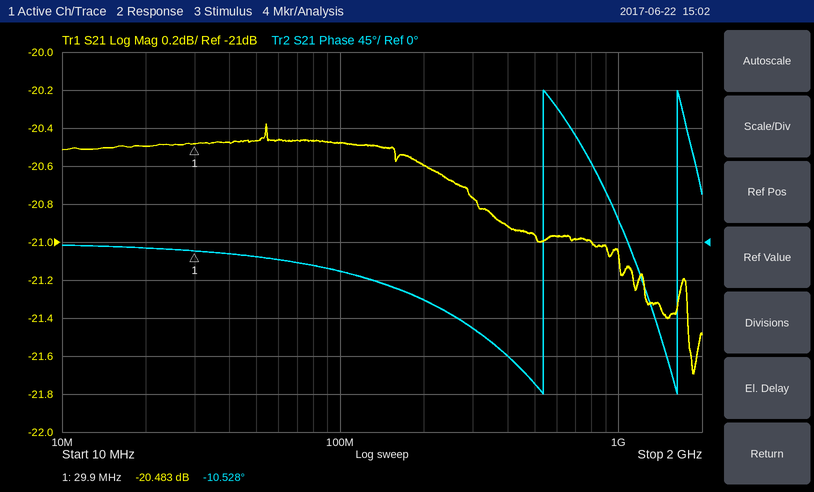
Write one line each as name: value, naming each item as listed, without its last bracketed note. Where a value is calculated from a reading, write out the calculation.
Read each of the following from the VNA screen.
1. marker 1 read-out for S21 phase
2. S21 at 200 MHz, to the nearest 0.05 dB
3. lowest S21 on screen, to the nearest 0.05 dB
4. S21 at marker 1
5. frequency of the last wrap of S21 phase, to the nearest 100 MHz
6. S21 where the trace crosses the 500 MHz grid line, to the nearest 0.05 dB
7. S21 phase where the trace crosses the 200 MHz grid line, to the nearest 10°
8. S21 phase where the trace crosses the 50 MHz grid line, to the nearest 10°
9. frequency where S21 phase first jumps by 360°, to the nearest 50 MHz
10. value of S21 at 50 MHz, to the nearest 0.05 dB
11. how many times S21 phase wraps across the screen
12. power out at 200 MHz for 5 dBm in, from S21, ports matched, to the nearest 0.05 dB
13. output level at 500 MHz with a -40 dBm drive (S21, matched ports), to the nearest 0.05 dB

marker 1 read-out for S21 phase: -10.528°
S21 at 200 MHz, to the nearest 0.05 dB: -20.60 dB
lowest S21 on screen, to the nearest 0.05 dB: -21.70 dB
S21 at marker 1: -20.483 dB
frequency of the last wrap of S21 phase, to the nearest 100 MHz: 1.6 GHz
S21 where the trace crosses the 500 MHz grid line, to the nearest 0.05 dB: -20.95 dB
S21 phase where the trace crosses the 200 MHz grid line, to the nearest 10°: -70°
S21 phase where the trace crosses the 50 MHz grid line, to the nearest 10°: -20°
frequency where S21 phase first jumps by 360°, to the nearest 50 MHz: 550 MHz
value of S21 at 50 MHz, to the nearest 0.05 dB: -20.45 dB
how many times S21 phase wraps across the screen: 2
power out at 200 MHz for 5 dBm in, from S21, ports matched, to the nearest 0.05 dB: 5 dBm + (-20.60 dB) = -15.60 dBm
output level at 500 MHz with a -40 dBm drive (S21, matched ports), to the nearest 0.05 dB: -40 dBm + (-20.95 dB) = -60.95 dBm
